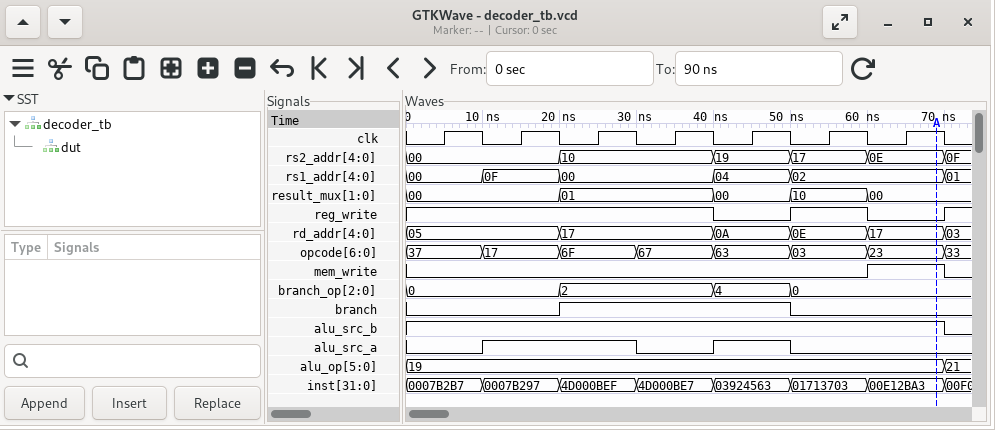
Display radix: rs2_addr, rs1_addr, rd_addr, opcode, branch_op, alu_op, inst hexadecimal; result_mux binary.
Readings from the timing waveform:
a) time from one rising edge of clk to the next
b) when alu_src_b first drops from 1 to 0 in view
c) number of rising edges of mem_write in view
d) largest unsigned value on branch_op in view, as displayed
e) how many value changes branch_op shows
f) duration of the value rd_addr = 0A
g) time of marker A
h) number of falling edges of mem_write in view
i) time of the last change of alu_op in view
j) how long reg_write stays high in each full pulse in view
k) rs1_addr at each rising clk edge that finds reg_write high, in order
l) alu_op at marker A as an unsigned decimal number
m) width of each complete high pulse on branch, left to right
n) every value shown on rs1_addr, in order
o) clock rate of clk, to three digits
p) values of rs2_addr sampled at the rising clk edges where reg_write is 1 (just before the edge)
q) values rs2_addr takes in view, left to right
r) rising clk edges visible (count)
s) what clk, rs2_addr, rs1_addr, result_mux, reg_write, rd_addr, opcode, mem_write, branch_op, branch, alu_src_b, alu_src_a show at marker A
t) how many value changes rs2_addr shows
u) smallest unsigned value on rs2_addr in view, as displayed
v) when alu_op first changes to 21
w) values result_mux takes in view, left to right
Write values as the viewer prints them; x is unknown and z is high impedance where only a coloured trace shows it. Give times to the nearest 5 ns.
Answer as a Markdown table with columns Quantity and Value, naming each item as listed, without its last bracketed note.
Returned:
| Quantity | Value |
|---|---|
| time from one rising edge of clk to the next | 10 ns |
| when alu_src_b first drops from 1 to 0 in view | 70 ns |
| number of rising edges of mem_write in view | 1 |
| largest unsigned value on branch_op in view, as displayed | 4 |
| how many value changes branch_op shows | 3 |
| duration of the value rd_addr = 0A | 10 ns |
| time of marker A | 70 ns |
| number of falling edges of mem_write in view | 1 |
| time of the last change of alu_op in view | 70 ns |
| how long reg_write stays high in each full pulse in view | 10 ns |
| rs1_addr at each rising clk edge that finds reg_write high, in order | 00, 0F, 00, 00, 02 |
| alu_op at marker A as an unsigned decimal number | 25 |
| width of each complete high pulse on branch, left to right | 30 ns |
| every value shown on rs1_addr, in order | 00, 0F, 00, 04, 02, 01 |
| clock rate of clk, to three digits | 100 MHz |
| values of rs2_addr sampled at the rising clk edges where reg_write is 1 | 00, 00, 10, 10, 17 |
| values rs2_addr takes in view, left to right | 00, 10, 19, 17, 0E, 0F |
| rising clk edges visible | 7 |
| what clk, rs2_addr, rs1_addr, result_mux, reg_write, rd_addr, opcode, mem_write, branch_op, branch, alu_src_b, alu_src_a show at marker A | clk=1, rs2_addr=0E, rs1_addr=02, result_mux=00, reg_write=0, rd_addr=17, opcode=23, mem_write=1, branch_op=0, branch=0, alu_src_b=1, alu_src_a=0 |
| how many value changes rs2_addr shows | 5 |
| smallest unsigned value on rs2_addr in view, as displayed | 00 |
| when alu_op first changes to 21 | 70 ns |
| values result_mux takes in view, left to right | 00, 01, 00, 10, 00 |
